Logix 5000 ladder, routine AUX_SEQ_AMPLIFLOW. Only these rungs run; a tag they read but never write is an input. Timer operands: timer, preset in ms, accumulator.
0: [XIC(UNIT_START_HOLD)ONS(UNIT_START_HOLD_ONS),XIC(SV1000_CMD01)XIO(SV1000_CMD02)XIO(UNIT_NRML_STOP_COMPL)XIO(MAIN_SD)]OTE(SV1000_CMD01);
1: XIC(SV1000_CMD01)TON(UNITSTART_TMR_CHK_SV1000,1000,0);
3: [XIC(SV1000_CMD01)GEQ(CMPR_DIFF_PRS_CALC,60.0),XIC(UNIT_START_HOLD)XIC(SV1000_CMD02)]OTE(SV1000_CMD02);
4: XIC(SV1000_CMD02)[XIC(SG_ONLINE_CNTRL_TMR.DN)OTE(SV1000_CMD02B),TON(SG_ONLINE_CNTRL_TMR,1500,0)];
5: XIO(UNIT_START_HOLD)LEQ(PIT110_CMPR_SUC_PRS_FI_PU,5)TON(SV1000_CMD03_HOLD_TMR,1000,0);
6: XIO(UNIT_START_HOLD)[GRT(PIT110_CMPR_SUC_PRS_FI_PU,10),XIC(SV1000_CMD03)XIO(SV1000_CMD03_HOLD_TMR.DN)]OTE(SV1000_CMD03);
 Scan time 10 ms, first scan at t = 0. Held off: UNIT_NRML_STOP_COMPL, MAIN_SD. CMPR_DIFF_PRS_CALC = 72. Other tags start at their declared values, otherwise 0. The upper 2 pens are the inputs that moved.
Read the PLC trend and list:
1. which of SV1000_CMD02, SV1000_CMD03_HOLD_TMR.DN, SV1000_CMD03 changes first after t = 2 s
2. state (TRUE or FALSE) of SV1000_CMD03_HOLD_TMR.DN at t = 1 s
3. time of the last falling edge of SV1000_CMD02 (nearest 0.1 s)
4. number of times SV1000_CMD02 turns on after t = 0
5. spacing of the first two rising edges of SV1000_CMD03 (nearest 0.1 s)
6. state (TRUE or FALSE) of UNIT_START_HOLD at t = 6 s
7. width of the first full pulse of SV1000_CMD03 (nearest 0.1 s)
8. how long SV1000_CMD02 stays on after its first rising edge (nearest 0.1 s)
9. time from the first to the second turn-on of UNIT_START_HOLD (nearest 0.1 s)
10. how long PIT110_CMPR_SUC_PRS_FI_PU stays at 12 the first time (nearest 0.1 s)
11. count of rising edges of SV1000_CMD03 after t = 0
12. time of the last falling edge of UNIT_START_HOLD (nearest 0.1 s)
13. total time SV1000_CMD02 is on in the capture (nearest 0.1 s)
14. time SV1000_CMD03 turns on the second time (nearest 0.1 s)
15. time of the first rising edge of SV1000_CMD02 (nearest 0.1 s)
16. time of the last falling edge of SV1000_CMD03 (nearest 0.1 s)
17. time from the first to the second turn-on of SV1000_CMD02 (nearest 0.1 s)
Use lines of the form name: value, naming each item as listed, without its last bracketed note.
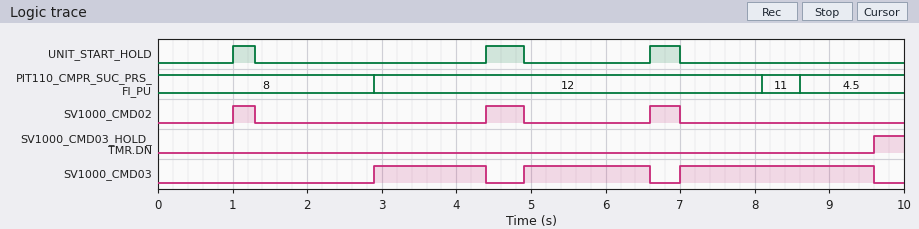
which of SV1000_CMD02, SV1000_CMD03_HOLD_TMR.DN, SV1000_CMD03 changes first after t = 2 s: SV1000_CMD03
state (TRUE or FALSE) of SV1000_CMD03_HOLD_TMR.DN at t = 1 s: FALSE
time of the last falling edge of SV1000_CMD02: 7.0 s
number of times SV1000_CMD02 turns on after t = 0: 3
spacing of the first two rising edges of SV1000_CMD03: 2.0 s
state (TRUE or FALSE) of UNIT_START_HOLD at t = 6 s: FALSE
width of the first full pulse of SV1000_CMD03: 1.5 s
how long SV1000_CMD02 stays on after its first rising edge: 0.3 s
time from the first to the second turn-on of UNIT_START_HOLD: 3.4 s
how long PIT110_CMPR_SUC_PRS_FI_PU stays at 12 the first time: 5.2 s
count of rising edges of SV1000_CMD03 after t = 0: 3
time of the last falling edge of UNIT_START_HOLD: 7.0 s
total time SV1000_CMD02 is on in the capture: 1.2 s
time SV1000_CMD03 turns on the second time: 4.9 s
time of the first rising edge of SV1000_CMD02: 1.0 s
time of the last falling edge of SV1000_CMD03: 9.6 s
time from the first to the second turn-on of SV1000_CMD02: 3.4 s
